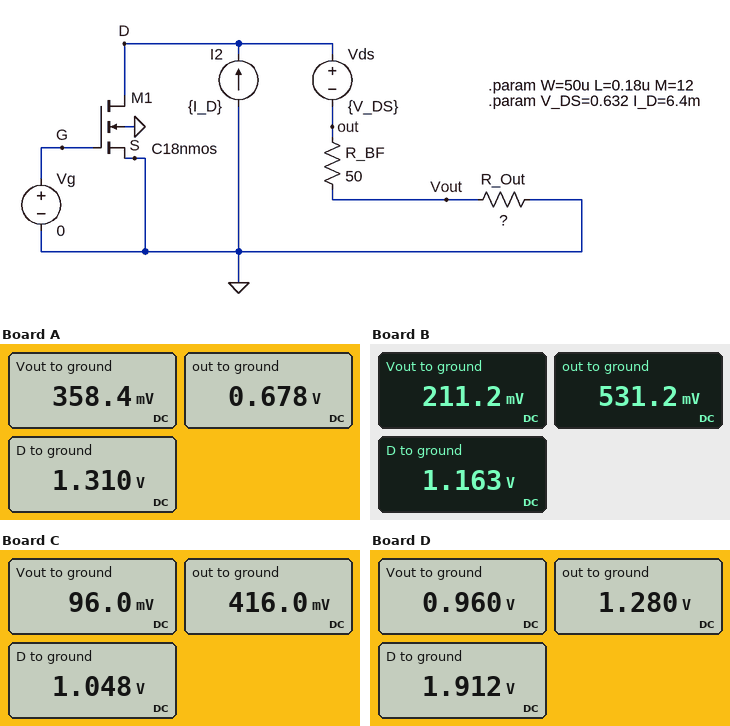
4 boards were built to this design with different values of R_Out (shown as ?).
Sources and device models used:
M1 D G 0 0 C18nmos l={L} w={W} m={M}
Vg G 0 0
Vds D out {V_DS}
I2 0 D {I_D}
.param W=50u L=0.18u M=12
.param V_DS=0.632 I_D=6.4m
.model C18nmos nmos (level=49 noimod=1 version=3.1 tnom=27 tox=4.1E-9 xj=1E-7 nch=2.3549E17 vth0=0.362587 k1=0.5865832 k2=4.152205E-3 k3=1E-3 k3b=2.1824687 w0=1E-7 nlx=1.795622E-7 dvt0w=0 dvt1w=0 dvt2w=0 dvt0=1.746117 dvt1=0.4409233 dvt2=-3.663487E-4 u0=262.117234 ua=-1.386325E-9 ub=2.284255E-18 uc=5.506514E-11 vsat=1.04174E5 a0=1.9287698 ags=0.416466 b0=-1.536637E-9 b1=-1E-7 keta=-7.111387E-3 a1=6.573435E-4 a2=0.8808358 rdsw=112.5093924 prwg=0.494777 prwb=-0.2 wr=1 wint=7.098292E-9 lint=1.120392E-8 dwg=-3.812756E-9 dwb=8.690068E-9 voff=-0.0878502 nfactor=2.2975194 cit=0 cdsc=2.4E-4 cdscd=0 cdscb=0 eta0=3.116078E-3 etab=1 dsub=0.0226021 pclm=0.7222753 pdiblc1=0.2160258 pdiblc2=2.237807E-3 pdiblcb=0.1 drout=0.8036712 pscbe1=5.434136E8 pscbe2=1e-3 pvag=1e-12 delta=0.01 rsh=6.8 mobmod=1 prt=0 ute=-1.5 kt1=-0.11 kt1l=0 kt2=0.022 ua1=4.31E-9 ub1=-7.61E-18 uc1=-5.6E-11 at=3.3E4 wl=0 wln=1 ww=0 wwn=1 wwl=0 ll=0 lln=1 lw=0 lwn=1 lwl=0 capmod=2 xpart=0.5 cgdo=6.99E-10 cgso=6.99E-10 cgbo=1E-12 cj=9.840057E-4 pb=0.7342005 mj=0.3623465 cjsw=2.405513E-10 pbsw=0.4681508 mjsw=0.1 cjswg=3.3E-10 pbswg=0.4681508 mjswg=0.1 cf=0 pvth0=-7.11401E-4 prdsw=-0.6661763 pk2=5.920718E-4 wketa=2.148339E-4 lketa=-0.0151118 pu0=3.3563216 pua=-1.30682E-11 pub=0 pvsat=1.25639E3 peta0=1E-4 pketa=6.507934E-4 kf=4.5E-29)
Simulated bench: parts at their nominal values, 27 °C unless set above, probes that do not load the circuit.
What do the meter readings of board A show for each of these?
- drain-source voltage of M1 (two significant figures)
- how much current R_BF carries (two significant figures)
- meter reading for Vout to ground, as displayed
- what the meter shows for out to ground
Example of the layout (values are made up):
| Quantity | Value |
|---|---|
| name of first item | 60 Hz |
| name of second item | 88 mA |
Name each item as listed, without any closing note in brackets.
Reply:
| Quantity | Value |
|---|---|
| drain-source voltage of M1 | 1.3 V |
| how much current R_BF carries | 6.4 mA |
| meter reading for Vout to ground, as displayed | 358.4 mV |
| what the meter shows for out to ground | 0.678 V |
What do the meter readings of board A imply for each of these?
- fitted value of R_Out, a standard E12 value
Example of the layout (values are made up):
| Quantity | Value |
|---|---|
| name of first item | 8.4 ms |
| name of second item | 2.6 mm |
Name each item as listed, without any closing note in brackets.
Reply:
| Quantity | Value |
|---|---|
| fitted value of R_Out, a standard E12 value | 56 Ω |
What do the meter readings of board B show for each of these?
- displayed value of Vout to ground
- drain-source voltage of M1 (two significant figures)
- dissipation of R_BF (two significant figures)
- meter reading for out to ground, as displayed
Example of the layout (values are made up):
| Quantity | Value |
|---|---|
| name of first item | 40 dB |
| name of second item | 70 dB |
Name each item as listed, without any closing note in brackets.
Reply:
| Quantity | Value |
|---|---|
| displayed value of Vout to ground | 211.2 mV |
| drain-source voltage of M1 | 1.2 V |
| dissipation of R_BF | 2.0 mW |
| meter reading for out to ground, as displayed | 531.2 mV |
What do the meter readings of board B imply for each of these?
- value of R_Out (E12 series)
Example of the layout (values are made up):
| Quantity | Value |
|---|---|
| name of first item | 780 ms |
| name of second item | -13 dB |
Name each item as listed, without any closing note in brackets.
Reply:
| Quantity | Value |
|---|---|
| value of R_Out | 33 Ω |
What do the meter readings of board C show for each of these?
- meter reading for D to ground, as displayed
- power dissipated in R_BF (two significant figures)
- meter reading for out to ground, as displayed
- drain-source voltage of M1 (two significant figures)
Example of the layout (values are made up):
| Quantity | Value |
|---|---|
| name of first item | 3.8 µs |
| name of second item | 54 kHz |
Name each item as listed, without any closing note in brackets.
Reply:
| Quantity | Value |
|---|---|
| meter reading for D to ground, as displayed | 1.048 V |
| power dissipated in R_BF | 2.0 mW |
| meter reading for out to ground, as displayed | 416.0 mV |
| drain-source voltage of M1 | 1.0 V |
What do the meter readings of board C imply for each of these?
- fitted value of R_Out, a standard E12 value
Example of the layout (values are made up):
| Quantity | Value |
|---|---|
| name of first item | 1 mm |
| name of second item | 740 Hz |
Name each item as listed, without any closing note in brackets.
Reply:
| Quantity | Value |
|---|---|
| fitted value of R_Out, a standard E12 value | 15 Ω |
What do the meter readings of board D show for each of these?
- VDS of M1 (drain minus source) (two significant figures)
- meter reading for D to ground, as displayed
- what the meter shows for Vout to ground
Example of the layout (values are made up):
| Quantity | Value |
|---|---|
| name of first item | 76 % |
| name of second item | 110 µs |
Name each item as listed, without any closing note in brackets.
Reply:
| Quantity | Value |
|---|---|
| VDS of M1 (drain minus source) | 1.9 V |
| meter reading for D to ground, as displayed | 1.912 V |
| what the meter shows for Vout to ground | 0.960 V |
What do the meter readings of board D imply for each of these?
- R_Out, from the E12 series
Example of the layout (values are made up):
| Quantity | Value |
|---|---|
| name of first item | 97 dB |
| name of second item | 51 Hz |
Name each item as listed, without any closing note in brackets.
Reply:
| Quantity | Value |
|---|---|
| R_Out, from the E12 series | 150 Ω |
